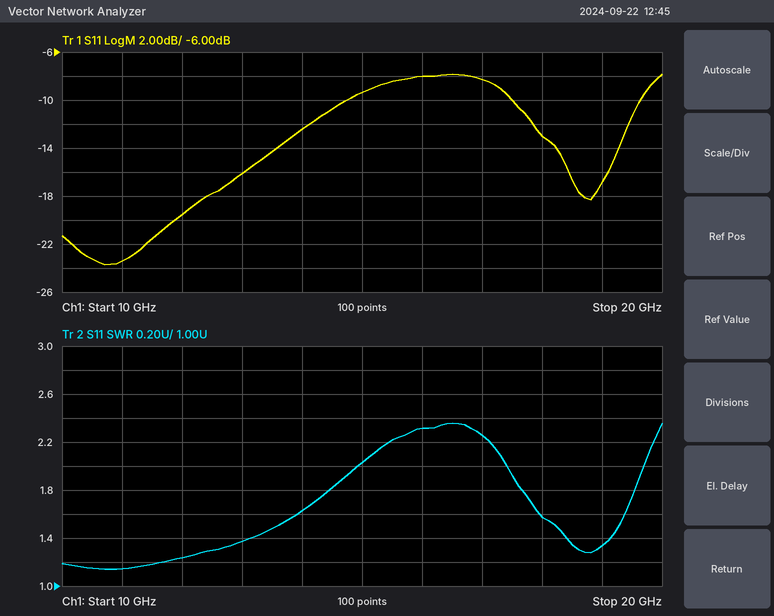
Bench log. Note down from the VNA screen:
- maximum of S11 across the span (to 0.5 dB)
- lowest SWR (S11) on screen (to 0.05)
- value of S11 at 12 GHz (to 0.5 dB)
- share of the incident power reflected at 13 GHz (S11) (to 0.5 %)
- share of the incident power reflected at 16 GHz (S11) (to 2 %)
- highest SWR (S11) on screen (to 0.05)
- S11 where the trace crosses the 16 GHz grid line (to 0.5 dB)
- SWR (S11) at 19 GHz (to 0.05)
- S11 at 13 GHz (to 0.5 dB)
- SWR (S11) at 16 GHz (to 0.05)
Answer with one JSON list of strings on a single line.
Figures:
["-8.0 dB", "1.15", "-19.5 dB", "2.5 %", "16 %", "2.35", "-8.0 dB", "1.35", "-16.0 dB", "2.30"]
